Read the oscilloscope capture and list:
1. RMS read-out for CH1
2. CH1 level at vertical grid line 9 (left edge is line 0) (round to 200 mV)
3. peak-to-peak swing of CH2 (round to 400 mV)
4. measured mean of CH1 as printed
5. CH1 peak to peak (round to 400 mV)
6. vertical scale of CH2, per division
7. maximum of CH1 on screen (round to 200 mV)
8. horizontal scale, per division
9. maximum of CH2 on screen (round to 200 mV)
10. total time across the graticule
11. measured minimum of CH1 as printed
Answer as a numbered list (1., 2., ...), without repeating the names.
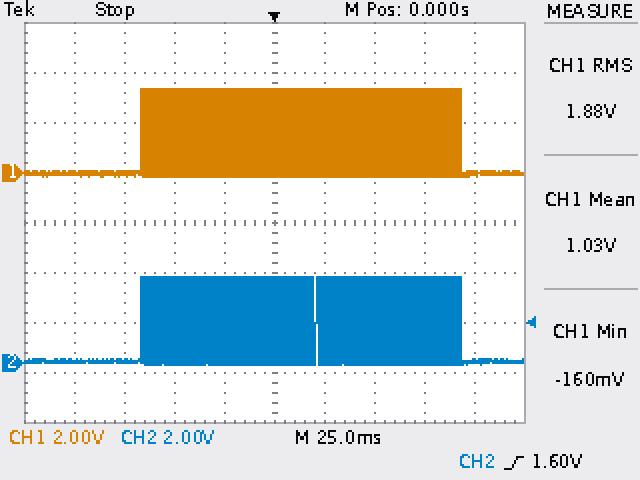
1. 1.88 V
2. 0.0 V
3. 3.6 V
4. 1.03 V
5. 3.6 V
6. 2 V
7. 3.4 V
8. 25 ms
9. 3.4 V
10. 250 ms
11. -160 mV
